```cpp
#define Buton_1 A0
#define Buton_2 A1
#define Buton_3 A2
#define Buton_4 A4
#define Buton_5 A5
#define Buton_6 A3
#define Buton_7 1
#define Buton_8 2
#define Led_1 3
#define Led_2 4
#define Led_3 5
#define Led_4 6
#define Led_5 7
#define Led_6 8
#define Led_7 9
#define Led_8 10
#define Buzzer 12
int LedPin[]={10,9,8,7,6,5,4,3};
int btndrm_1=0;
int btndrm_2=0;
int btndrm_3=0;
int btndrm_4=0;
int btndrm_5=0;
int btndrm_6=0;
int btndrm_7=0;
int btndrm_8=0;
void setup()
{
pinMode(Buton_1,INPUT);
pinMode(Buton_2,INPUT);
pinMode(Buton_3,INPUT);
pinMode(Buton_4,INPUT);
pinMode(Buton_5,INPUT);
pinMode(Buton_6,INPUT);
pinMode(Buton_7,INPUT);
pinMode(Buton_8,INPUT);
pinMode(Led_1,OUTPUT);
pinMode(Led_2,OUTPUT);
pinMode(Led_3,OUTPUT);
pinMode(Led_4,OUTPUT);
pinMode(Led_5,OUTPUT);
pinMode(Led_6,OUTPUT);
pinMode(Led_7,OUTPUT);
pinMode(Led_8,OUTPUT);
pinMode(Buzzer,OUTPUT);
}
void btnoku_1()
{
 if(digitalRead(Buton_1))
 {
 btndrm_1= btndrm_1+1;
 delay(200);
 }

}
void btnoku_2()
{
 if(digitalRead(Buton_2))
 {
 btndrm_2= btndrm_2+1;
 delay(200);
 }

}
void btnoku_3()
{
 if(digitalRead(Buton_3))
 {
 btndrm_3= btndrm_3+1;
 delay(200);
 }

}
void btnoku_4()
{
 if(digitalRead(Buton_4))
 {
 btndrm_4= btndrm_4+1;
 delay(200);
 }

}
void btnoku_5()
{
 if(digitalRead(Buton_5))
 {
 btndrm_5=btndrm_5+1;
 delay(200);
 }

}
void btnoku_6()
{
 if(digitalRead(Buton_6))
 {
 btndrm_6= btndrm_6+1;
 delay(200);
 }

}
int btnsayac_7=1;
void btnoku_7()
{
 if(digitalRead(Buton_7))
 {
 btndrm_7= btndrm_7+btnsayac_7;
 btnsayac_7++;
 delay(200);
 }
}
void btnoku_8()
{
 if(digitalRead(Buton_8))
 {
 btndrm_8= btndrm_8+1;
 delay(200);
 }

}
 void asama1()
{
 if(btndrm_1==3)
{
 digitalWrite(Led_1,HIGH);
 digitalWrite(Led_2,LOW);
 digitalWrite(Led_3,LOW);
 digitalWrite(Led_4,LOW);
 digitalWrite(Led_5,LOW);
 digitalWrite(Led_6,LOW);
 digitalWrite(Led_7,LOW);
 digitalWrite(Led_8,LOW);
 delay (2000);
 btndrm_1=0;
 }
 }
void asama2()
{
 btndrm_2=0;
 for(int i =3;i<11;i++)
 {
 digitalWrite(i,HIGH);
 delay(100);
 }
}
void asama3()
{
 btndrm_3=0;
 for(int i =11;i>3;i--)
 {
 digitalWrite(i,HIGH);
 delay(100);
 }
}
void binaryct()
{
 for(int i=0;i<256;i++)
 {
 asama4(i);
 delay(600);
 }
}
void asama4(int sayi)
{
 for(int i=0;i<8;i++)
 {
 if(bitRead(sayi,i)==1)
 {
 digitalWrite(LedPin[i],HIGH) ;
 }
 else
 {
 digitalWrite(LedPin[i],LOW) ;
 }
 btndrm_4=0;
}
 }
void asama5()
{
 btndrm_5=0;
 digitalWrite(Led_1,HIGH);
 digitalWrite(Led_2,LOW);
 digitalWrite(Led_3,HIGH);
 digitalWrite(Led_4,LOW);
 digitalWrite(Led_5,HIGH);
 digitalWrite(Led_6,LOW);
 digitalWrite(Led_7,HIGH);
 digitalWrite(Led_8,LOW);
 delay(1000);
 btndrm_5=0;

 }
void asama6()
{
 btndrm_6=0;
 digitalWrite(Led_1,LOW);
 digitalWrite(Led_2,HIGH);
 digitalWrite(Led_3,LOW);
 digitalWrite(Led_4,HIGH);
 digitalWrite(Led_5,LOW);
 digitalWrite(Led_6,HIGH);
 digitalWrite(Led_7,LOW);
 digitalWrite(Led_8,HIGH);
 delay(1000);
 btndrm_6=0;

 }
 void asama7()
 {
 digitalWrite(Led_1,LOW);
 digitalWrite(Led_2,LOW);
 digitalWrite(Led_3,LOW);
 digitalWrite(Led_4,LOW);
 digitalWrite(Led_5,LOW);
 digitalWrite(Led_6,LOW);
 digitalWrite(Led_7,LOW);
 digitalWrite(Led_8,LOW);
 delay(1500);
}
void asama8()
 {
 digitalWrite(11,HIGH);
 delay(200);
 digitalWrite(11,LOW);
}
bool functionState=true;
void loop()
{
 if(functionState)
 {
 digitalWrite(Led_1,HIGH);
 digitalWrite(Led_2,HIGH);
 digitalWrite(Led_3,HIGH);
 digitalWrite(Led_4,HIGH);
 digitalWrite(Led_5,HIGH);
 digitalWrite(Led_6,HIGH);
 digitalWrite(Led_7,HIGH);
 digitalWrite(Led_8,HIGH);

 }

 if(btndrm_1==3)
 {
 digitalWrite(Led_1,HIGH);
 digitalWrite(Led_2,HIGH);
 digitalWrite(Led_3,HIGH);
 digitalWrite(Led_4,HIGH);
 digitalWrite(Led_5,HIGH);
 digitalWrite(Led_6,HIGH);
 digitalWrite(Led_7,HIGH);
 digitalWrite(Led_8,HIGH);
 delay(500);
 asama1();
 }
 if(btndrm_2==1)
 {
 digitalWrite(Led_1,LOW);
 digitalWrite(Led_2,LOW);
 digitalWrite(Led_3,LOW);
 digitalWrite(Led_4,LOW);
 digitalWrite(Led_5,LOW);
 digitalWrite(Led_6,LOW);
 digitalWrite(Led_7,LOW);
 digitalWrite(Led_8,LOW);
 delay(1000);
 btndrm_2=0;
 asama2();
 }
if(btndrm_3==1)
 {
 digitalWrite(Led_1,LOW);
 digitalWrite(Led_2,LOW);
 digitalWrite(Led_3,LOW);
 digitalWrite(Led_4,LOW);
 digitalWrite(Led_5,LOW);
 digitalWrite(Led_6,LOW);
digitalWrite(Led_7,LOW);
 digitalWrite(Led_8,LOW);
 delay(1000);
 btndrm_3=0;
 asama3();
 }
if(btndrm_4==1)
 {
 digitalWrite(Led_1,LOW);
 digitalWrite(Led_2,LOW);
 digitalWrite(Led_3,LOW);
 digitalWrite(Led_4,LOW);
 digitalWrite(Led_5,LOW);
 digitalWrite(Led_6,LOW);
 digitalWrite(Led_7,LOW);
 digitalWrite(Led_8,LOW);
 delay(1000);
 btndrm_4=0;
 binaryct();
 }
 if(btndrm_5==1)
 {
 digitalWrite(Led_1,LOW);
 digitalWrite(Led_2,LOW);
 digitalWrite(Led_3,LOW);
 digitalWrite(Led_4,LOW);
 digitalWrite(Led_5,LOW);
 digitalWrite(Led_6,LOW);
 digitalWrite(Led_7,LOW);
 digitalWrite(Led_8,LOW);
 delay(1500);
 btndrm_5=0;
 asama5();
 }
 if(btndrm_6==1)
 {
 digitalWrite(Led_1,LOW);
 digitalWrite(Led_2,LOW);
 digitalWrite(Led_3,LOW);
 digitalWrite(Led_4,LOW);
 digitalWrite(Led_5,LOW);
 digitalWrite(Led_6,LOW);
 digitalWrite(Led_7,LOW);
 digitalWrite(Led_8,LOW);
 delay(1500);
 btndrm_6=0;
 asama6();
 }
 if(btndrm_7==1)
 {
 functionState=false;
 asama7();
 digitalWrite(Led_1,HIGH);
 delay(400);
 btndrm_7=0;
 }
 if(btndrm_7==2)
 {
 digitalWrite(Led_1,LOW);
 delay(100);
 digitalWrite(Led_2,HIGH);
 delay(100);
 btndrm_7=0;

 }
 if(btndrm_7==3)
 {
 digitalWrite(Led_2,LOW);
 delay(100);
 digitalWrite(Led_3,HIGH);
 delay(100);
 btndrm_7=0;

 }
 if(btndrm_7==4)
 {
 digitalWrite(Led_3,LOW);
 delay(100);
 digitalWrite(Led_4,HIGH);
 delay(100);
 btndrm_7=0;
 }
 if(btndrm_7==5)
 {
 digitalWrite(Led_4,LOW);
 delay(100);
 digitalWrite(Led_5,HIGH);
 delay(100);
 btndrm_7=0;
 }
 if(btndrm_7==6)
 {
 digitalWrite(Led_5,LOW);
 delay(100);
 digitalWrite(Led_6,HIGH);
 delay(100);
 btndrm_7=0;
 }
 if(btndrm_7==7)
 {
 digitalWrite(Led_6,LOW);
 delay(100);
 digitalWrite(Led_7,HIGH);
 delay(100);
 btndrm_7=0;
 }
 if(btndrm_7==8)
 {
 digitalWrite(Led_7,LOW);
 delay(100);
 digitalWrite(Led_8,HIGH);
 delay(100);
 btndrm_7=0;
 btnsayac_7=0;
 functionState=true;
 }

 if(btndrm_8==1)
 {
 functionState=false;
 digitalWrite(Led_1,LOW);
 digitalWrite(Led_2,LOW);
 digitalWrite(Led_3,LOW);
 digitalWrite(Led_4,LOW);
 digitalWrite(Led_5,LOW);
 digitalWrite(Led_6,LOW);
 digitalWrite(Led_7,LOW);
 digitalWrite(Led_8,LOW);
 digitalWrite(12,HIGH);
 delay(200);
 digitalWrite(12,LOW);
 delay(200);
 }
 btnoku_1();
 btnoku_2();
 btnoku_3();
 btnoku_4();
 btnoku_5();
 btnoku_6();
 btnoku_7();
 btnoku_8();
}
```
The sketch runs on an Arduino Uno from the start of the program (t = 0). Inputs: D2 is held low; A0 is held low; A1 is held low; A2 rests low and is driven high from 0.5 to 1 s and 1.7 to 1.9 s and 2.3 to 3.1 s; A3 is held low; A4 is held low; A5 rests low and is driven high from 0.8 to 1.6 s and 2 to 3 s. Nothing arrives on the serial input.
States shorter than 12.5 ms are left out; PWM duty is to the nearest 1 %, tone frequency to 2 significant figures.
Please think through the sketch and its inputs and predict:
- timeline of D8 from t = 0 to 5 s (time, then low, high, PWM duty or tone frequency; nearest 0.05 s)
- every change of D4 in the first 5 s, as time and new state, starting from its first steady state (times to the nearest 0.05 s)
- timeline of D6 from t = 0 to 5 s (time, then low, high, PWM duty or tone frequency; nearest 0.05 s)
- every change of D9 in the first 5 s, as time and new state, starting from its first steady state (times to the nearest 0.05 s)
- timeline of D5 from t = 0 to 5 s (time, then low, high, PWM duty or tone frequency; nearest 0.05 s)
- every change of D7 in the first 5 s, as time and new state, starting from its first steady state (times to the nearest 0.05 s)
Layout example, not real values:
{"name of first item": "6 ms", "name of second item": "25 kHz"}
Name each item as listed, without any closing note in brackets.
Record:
{"timeline of D8 from t = 0 to 5 s": "0 s high; 0.7 s low; 2 s high; 2.9 s low; 4.2 s high; 4.7 s low", "every change of D4 in the first 5 s, as time and new state, starting from its first steady state": "0 s high; 0.7 s low; 2.4 s high; 2.9 s low; 4.6 s high; 4.7 s low", "timeline of D6 from t = 0 to 5 s": "0 s high; 0.7 s low; 2.2 s high; 2.9 s low; 4.4 s high; 4.7 s low", "every change of D9 in the first 5 s, as time and new state, starting from its first steady state": "0 s high; 0.7 s low; 1.9 s high; 2.9 s low; 4.1 s high; 4.7 s low", "timeline of D5 from t = 0 to 5 s": "0 s high; 0.7 s low; 2.3 s high; 2.9 s low; 4.5 s high; 4.7 s low", "every change of D7 in the first 5 s, as time and new state, starting from its first steady state": "0 s high; 0.7 s low; 2.1 s high; 2.9 s low; 4.3 s high; 4.7 s low"}
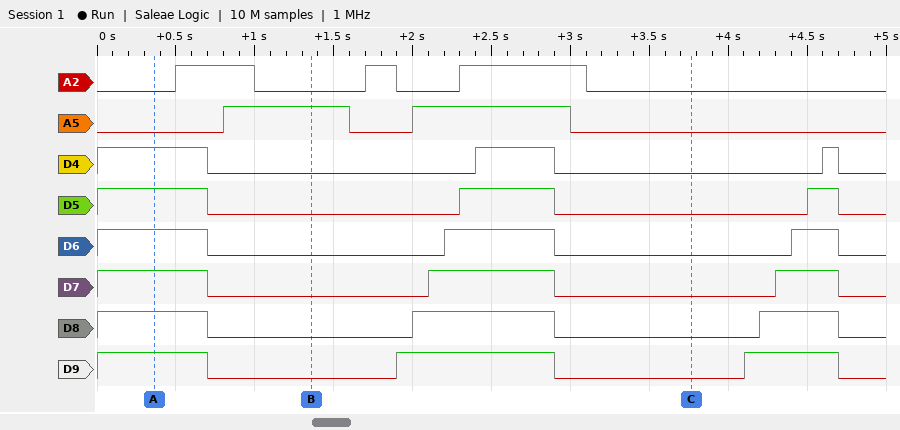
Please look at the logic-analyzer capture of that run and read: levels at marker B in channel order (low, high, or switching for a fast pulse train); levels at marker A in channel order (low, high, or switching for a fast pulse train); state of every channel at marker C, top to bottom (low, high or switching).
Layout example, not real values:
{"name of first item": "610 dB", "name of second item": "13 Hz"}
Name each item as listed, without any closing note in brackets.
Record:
{"levels at marker B in channel order": "A2 low, A5 high, D4 low, D5 low, D6 low, D7 low, D8 low, D9 low", "levels at marker A in channel order": "A2 low, A5 low, D4 high, D5 high, D6 high, D7 high, D8 high, D9 high", "state of every channel at marker C, top to bottom": "A2 low, A5 low, D4 low, D5 low, D6 low, D7 low, D8 low, D9 low"}
